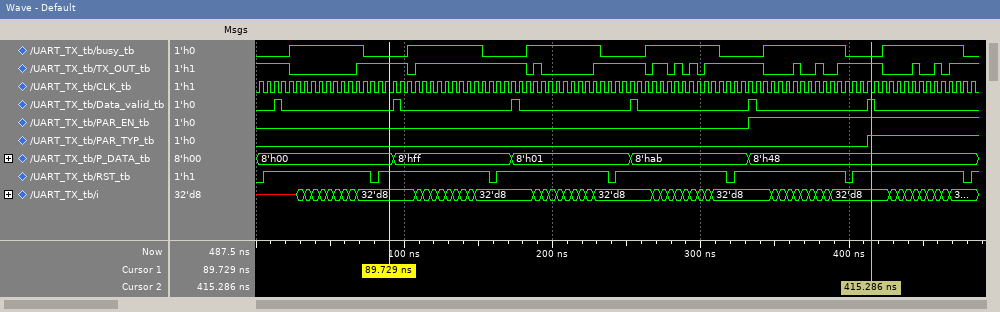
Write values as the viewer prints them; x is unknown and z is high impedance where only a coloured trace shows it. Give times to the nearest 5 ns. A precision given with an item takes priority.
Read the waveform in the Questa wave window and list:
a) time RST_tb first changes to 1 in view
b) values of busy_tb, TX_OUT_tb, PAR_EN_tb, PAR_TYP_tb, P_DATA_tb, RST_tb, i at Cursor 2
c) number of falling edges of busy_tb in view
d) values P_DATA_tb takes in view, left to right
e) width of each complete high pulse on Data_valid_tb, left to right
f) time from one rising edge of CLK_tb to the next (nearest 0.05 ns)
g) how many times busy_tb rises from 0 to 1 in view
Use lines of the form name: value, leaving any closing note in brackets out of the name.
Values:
time RST_tb first changes to 1 in view: 5 ns
values of busy_tb, TX_OUT_tb, PAR_EN_tb, PAR_TYP_tb, P_DATA_tb, RST_tb, i at Cursor 2: busy_tb=0, TX_OUT_tb=1, PAR_EN_tb=1, PAR_TYP_tb=1, P_DATA_tb=8'h48, RST_tb=1, i=32'd8
number of falling edges of busy_tb in view: 6
values P_DATA_tb takes in view, left to right: 8'h00, 8'hff, 8'h01, 8'hab, 8'h48
width of each complete high pulse on Data_valid_tb, left to right: 5 ns, 5 ns, 5 ns, 5 ns, 5 ns, 5 ns
time from one rising edge of CLK_tb to the next: 5 ns
how many times busy_tb rises from 0 to 1 in view: 6
